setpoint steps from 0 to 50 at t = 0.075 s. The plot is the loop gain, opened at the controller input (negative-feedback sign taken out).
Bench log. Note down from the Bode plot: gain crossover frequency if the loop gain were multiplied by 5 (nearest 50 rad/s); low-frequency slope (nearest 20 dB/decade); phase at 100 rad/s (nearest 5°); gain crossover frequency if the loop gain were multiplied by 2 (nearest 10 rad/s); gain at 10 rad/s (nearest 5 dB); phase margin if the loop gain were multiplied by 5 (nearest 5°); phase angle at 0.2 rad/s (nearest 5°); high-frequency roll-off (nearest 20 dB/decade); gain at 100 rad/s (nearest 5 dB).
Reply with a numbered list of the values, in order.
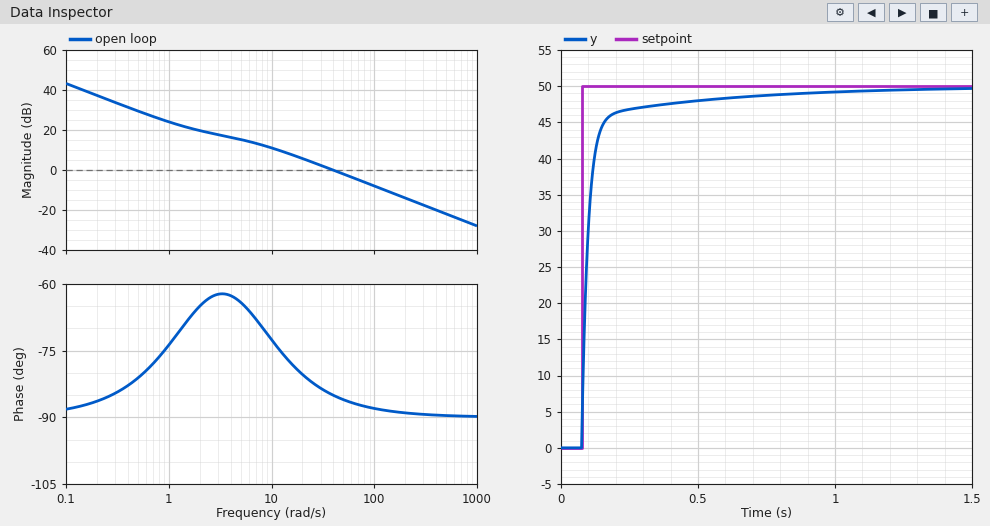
1. 200 rad/s
2. -20 dB/decade
3. -90°
4. 80 rad/s
5. 10 dB
6. 90°
7. -85°
8. -20 dB/decade
9. -10 dB
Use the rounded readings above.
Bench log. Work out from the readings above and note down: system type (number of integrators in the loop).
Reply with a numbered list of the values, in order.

1. 1
